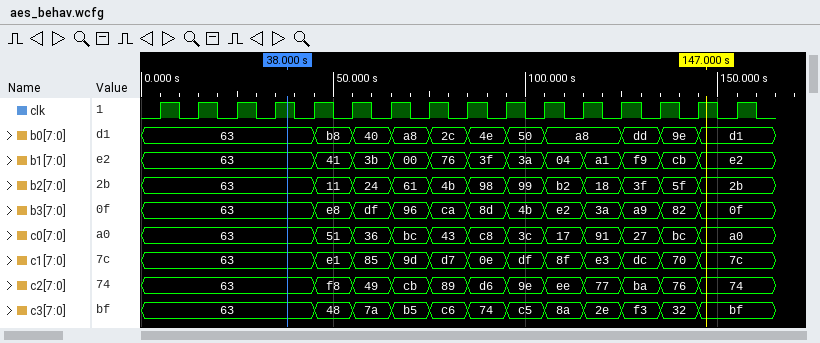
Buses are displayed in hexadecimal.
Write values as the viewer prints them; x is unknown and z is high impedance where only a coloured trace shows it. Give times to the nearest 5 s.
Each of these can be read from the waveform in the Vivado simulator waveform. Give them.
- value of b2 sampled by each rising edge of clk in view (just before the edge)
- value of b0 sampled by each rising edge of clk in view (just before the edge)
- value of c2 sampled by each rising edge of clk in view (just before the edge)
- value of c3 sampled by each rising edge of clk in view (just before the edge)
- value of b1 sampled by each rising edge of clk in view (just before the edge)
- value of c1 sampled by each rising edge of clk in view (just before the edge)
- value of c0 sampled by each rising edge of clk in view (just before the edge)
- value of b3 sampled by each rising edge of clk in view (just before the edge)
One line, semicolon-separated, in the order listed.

63, 63, 63, 63, 63, 11, 24, 61, 4b, 98, 99, b2, 18, 3f, 5f, 2b; 63, 63, 63, 63, 63, b8, 40, a8, 2c, 4e, 50, a8, a8, dd, 9e, d1; 63, 63, 63, 63, 63, f8, 49, cb, 89, d6, 9e, ee, 77, ba, 76, 74; 63, 63, 63, 63, 63, 48, 7a, b5, c6, 74, c5, 8a, 2e, f3, 32, bf; 63, 63, 63, 63, 63, 41, 3b, 00, 76, 3f, 3a, 04, a1, f9, cb, e2; 63, 63, 63, 63, 63, e1, 85, 9d, d7, 0e, df, 8f, e3, dc, 70, 7c; 63, 63, 63, 63, 63, 51, 36, bc, 43, c8, 3c, 17, 91, 27, bc, a0; 63, 63, 63, 63, 63, e8, df, 96, ca, 8d, 4b, e2, 3a, a9, 82, 0f
